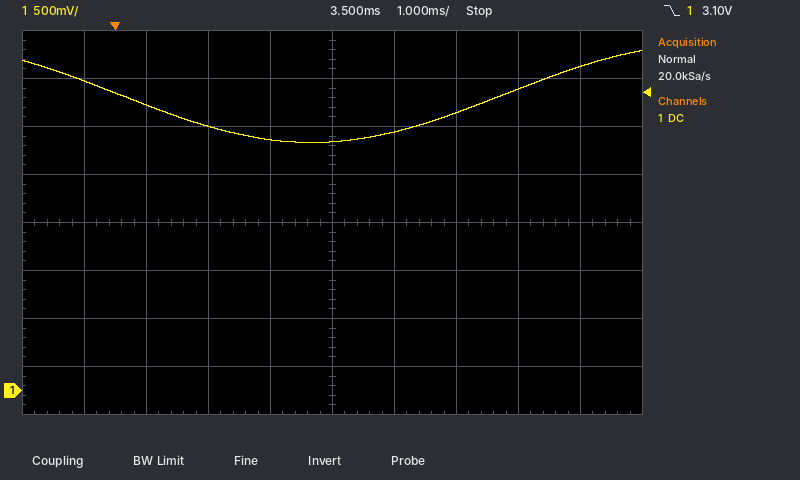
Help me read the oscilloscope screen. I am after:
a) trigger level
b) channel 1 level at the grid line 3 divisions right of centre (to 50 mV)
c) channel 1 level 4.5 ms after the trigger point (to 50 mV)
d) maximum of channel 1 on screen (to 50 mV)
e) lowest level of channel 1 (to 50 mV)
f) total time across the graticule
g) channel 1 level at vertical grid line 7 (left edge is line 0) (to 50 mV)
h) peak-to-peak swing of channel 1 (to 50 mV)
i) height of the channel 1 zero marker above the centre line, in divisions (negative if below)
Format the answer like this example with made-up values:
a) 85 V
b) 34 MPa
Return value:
a) 3.10 V
b) 3.15 V
c) 2.70 V
d) 3.55 V
e) 2.60 V
f) 10 ms
g) 2.90 V
h) 950 mV
i) -3.5 div
